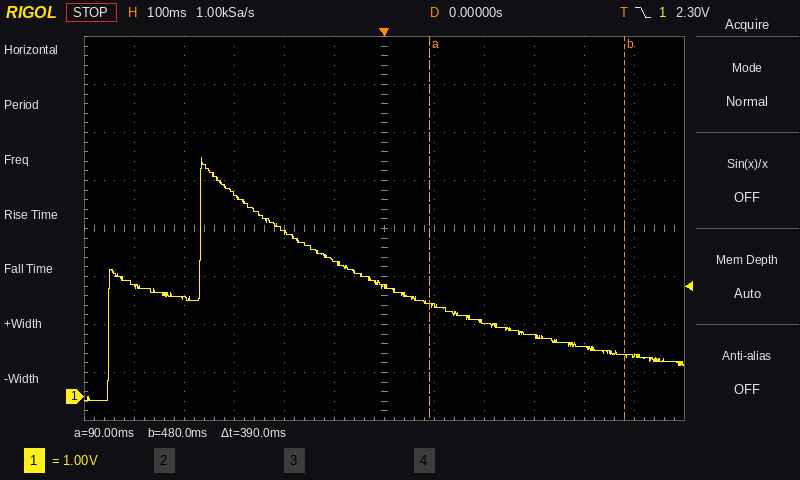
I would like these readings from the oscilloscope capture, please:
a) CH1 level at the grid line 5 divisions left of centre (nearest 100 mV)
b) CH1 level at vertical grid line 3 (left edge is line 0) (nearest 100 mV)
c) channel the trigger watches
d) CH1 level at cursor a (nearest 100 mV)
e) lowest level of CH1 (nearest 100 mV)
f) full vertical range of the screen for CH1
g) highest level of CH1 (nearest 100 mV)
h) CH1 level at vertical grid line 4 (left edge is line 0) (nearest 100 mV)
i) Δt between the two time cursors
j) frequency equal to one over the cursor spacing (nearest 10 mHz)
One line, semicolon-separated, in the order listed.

2.3 V; 4.2 V; CH1; 1.9 V; -100 mV; 8 V; 5.0 V; 3.4 V; 390 ms; 2.56 Hz
